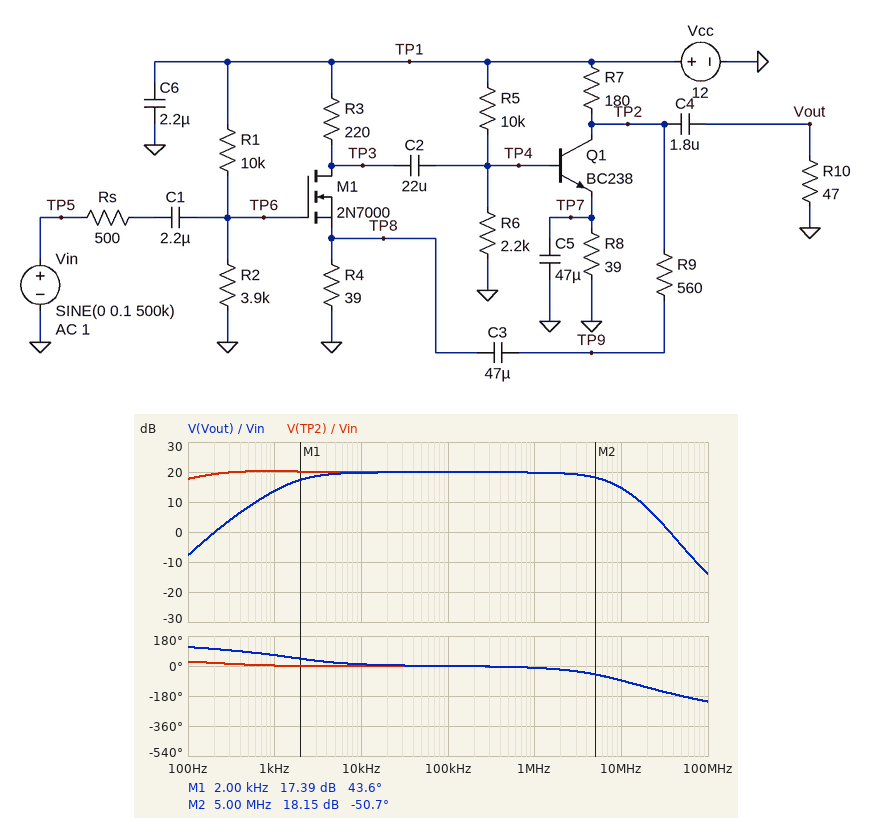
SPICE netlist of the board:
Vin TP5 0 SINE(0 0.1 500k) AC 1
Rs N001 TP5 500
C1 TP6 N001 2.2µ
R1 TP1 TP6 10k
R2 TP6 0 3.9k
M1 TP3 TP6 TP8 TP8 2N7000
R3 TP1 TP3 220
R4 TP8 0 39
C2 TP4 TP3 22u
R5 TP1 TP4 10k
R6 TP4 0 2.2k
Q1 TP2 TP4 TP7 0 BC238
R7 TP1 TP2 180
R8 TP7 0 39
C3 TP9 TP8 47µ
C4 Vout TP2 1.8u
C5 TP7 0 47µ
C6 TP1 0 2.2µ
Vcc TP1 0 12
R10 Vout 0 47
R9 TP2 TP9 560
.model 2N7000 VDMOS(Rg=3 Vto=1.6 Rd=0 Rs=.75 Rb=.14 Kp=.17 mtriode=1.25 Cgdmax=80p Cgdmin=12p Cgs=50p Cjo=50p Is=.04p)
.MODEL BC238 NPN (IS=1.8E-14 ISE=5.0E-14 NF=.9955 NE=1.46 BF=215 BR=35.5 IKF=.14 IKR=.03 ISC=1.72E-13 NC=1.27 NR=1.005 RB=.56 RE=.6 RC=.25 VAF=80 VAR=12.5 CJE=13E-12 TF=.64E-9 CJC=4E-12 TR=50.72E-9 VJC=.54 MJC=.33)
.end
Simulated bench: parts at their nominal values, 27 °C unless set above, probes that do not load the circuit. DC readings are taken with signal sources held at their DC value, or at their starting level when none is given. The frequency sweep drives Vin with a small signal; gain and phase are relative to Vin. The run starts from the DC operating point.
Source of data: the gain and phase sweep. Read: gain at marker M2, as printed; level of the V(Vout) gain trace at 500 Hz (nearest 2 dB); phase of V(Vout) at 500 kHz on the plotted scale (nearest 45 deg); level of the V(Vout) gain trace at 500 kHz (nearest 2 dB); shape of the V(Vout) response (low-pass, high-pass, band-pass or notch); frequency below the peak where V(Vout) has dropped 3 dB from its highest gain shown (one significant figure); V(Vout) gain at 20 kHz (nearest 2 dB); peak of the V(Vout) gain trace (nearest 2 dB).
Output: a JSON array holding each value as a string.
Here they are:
["18.15 dB", "8 dB", "0 deg", "20 dB", "band-pass", "2 kHz", "20 dB", "20 dB"]
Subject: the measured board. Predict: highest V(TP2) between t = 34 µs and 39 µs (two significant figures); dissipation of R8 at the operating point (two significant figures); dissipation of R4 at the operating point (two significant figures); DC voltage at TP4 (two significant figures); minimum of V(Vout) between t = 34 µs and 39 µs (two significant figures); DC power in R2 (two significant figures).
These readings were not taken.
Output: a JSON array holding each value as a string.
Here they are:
["7.8 V", "32 mW", "34 mW", "1.9 V", "-990 mV", "2.9 mW"]
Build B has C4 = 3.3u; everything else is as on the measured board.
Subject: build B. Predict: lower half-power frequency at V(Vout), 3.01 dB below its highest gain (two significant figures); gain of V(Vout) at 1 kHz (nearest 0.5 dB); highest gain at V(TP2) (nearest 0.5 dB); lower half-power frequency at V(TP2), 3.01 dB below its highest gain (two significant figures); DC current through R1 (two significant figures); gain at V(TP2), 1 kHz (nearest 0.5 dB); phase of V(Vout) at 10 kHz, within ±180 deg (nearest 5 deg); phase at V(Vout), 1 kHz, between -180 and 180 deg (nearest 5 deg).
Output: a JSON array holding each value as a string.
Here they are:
["1.1 kHz", "16.5 dB", "20.0 dB", "80 Hz", "860 µA", "19.5 dB", "5 deg", "50 deg"]
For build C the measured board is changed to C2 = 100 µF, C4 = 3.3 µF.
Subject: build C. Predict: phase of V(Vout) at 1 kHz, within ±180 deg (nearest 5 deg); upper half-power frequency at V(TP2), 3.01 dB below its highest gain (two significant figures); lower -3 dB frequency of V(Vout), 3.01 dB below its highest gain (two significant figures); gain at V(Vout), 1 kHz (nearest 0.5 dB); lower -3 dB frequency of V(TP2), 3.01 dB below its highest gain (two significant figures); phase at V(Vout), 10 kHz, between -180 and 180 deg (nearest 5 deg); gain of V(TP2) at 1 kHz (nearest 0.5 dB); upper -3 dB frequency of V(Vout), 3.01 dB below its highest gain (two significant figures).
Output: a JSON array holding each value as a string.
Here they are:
["50 deg", "6.9 MHz", "1.1 kHz", "16.5 dB", "80 Hz", "5 deg", "19.5 dB", "6.9 MHz"]
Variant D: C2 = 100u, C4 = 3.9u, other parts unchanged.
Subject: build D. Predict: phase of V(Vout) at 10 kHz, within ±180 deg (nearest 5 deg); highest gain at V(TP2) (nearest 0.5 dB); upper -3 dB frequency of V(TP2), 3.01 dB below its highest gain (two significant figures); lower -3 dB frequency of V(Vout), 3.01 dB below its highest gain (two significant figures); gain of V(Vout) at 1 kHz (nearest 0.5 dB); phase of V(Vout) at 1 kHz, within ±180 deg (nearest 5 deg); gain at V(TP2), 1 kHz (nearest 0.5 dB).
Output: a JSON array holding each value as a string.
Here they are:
["5 deg", "20.0 dB", "6.9 MHz", "950 Hz", "17.0 dB", "45 deg", "19.5 dB"]
